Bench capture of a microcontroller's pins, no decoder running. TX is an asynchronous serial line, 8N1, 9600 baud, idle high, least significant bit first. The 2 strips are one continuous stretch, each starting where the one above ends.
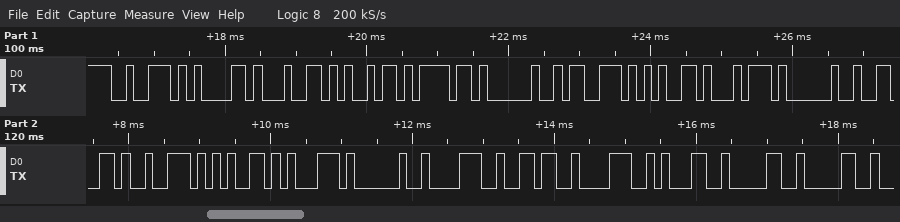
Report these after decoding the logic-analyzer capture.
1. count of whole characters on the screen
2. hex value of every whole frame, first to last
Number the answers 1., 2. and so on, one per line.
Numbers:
1. 21
2. 0x72 0x61 0x64 0x69 0x6F 0x20 0x73 0x65 0x74 0x20 0x66 0x72 0x65 0x71 0x20 0x38 0x36 0x38 0x31 0x30 0x30
